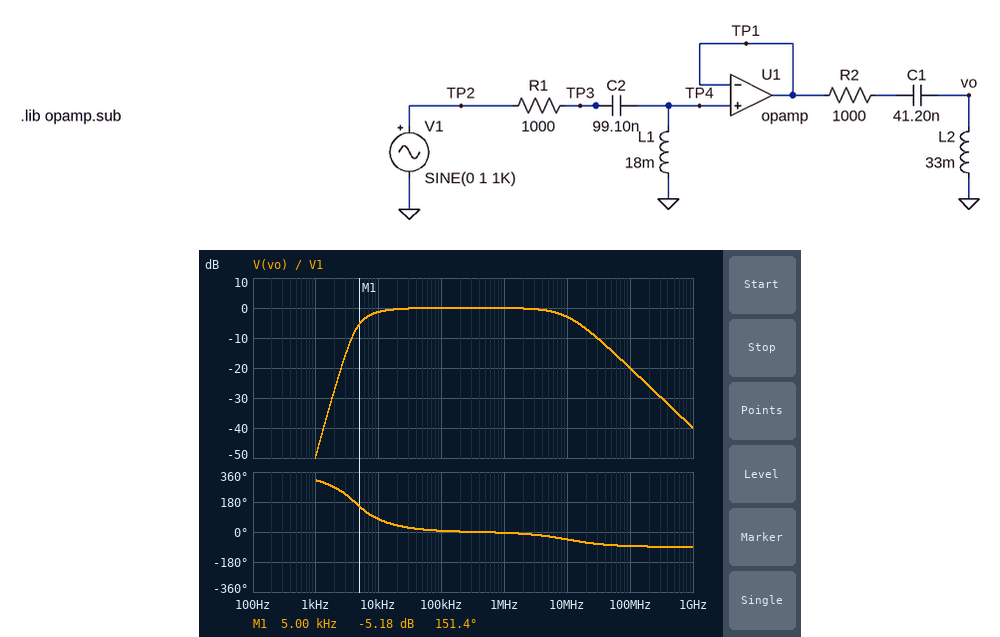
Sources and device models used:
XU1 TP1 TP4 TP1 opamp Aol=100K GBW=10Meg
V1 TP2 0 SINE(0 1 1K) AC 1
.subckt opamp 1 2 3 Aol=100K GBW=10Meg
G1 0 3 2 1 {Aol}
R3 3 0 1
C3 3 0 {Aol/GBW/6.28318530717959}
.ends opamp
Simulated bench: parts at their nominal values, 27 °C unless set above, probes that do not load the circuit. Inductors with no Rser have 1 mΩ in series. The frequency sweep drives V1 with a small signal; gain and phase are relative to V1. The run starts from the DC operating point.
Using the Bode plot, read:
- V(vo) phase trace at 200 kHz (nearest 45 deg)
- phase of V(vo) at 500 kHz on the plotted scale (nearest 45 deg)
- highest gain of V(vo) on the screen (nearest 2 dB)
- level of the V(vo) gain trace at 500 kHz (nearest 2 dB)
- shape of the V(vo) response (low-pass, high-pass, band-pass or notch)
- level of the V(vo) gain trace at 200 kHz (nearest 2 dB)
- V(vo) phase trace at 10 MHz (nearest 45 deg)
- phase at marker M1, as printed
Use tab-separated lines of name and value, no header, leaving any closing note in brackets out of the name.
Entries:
V(vo) phase trace at 200 kHz	0 deg
phase of V(vo) at 500 kHz on the plotted scale	0 deg
highest gain of V(vo) on the screen	0 dB
level of the V(vo) gain trace at 500 kHz	0 dB
shape of the V(vo) response	band-pass
level of the V(vo) gain trace at 200 kHz	0 dB
V(vo) phase trace at 10 MHz	-45 deg
phase at marker M1, as printed	151.4 deg
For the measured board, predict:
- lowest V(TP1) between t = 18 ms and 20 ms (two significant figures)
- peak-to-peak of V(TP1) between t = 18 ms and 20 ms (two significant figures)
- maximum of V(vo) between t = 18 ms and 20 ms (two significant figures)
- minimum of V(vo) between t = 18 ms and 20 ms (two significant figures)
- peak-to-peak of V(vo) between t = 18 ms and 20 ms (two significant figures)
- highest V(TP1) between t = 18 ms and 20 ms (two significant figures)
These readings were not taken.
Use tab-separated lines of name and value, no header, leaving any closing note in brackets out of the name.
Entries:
lowest V(TP1) between t = 18 ms and 20 ms	-63 mV
peak-to-peak of V(TP1) between t = 18 ms and 20 ms	130 mV
maximum of V(vo) between t = 18 ms and 20 ms	3.4 mV
minimum of V(vo) between t = 18 ms and 20 ms	-3.4 mV
peak-to-peak of V(vo) between t = 18 ms and 20 ms	6.9 mV
highest V(TP1) between t = 18 ms and 20 ms	63 mV
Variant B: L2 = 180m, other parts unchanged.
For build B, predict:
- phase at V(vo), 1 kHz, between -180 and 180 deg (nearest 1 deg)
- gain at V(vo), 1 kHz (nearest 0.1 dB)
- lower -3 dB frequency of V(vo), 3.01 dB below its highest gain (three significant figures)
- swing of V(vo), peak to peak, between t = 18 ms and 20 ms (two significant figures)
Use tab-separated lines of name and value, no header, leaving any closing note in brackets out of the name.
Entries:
phase at V(vo), 1 kHz, between -180 and 180 deg	-54 deg
gain at V(vo), 1 kHz	-32.2 dB
lower -3 dB frequency of V(vo), 3.01 dB below its highest gain	6.41 kHz
swing of V(vo), peak to peak, between t = 18 ms and 20 ms	49 mV
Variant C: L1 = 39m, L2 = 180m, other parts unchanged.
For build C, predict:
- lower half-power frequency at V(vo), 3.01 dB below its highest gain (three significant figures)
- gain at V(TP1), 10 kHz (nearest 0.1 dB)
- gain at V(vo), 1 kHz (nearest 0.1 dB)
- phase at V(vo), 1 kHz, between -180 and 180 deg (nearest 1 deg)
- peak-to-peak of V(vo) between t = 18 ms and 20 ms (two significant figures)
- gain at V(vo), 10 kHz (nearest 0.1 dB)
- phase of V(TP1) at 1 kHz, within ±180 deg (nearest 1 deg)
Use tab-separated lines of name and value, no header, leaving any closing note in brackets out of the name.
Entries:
lower half-power frequency at V(vo), 3.01 dB below its highest gain	1.76 kHz
gain at V(TP1), 10 kHz	-0.2 dB
gain at V(vo), 1 kHz	-25.0 dB
phase at V(vo), 1 kHz, between -180 and 180 deg	-56 deg
peak-to-peak of V(vo) between t = 18 ms and 20 ms	110 mV
gain at V(vo), 10 kHz	0.1 dB
phase of V(TP1) at 1 kHz, within ±180 deg	144 deg
